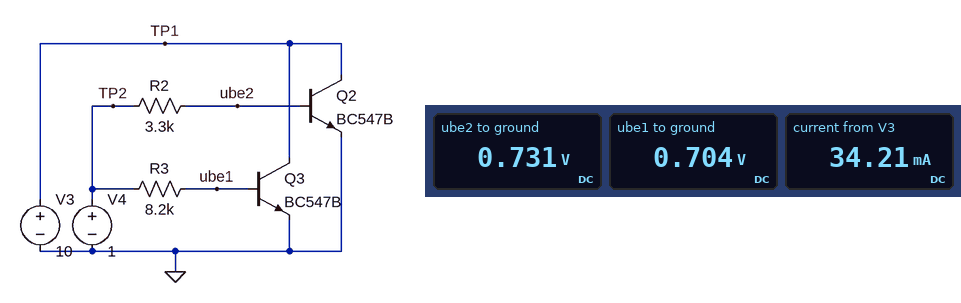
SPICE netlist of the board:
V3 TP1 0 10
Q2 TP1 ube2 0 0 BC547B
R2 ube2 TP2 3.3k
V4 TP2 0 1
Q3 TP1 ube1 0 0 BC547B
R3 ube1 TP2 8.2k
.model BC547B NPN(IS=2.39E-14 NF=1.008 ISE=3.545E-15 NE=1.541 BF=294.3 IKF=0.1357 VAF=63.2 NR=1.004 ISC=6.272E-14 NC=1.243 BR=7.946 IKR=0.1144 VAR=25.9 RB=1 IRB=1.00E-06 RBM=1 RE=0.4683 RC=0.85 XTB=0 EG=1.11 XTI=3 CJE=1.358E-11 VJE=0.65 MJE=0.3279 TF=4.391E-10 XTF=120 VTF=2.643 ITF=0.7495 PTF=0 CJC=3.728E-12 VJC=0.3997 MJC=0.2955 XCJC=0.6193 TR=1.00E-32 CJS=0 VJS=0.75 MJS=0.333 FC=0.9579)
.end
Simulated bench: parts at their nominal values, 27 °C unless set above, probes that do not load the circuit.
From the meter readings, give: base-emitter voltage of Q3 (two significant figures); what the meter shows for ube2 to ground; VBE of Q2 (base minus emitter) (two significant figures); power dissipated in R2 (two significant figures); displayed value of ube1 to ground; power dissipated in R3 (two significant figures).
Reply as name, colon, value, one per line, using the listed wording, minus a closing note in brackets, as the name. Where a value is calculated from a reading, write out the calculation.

base-emitter voltage of Q3: 704 mV = 700 mV
what the meter shows for ube2 to ground: 0.731 V
VBE of Q2 (base minus emitter): 731 mV = 730 mV
power dissipated in R2: (1 V - 731 mV)^2 / 3.3 kΩ = 22 µW
displayed value of ube1 to ground: 0.704 V
power dissipated in R3: (1 V - 704 mV)^2 / 8.2 kΩ = 11 µW
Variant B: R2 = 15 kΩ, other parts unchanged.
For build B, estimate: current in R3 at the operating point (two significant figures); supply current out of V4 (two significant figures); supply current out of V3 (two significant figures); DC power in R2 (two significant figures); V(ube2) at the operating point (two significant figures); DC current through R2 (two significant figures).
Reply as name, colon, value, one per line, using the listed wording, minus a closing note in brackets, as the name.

current in R3 at the operating point: 36 µA
supply current out of V4: 57 µA
supply current out of V3: 18 mA
DC power in R2: 6.5 µW
V(ube2) at the operating point: 690 mV
DC current through R2: 21 µA
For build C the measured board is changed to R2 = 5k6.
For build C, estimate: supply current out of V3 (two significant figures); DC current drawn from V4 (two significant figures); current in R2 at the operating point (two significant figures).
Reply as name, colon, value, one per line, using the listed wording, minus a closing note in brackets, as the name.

supply current out of V3: 26 mA
DC current drawn from V4: 87 µA
current in R2 at the operating point: 51 µA
